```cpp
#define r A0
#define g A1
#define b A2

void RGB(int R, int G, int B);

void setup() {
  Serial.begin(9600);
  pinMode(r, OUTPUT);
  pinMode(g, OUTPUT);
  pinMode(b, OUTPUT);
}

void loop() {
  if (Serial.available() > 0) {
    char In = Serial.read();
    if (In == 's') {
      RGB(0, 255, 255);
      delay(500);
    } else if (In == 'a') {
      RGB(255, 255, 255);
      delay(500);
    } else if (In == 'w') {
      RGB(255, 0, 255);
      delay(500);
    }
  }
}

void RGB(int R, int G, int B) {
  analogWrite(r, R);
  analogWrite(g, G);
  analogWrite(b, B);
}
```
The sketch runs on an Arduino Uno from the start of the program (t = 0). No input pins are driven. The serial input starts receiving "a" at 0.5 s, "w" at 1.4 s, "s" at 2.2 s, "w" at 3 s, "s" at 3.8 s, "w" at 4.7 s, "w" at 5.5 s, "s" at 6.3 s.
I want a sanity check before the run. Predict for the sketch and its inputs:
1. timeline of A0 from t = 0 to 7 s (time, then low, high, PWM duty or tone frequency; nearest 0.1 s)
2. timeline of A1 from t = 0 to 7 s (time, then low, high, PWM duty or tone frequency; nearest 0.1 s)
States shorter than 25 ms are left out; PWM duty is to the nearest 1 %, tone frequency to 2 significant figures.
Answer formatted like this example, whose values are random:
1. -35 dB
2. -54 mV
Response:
1. 0 s low; 0.5 s high; 2.2 s low; 3 s high; 3.8 s low; 4.7 s high; 6.3 s low
2. 0 s low; 0.5 s high; 1.4 s low; 2.2 s high; 3 s low; 3.8 s high; 4.7 s low; 6.3 s high
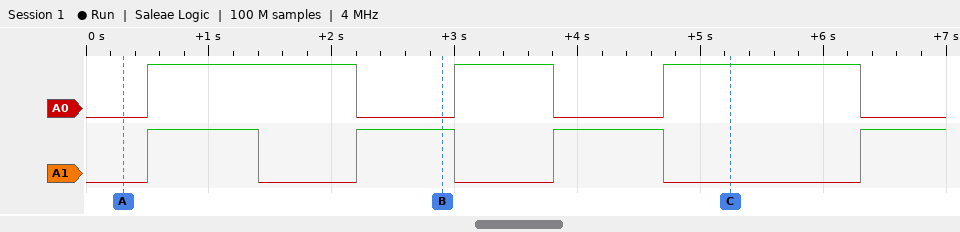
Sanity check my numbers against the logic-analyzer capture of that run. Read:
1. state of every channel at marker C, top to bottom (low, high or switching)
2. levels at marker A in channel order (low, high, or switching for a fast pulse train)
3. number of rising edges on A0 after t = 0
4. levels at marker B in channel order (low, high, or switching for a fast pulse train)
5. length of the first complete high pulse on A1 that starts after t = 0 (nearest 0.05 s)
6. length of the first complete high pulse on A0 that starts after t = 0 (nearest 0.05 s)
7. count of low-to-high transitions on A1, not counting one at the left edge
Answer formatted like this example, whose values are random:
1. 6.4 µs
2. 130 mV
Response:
1. A0 high, A1 low
2. A0 low, A1 low
3. 3
4. A0 low, A1 high
5. 0.90 s
6. 1.70 s
7. 4
